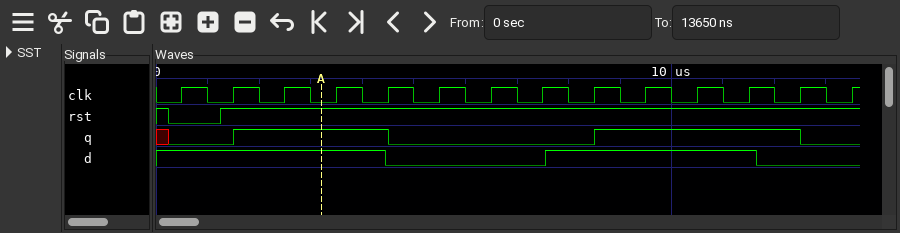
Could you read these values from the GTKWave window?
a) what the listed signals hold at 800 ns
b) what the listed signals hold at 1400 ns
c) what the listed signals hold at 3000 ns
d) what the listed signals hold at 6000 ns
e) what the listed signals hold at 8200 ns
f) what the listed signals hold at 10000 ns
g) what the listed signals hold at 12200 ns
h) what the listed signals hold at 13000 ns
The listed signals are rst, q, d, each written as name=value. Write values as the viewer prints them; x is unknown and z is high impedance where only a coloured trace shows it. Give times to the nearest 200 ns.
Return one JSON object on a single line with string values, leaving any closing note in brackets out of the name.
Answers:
{"what the listed signals hold at 800 ns": "rst=0, q=0, d=1", "what the listed signals hold at 1400 ns": "rst=1, q=0, d=1", "what the listed signals hold at 3000 ns": "rst=1, q=1, d=1", "what the listed signals hold at 6000 ns": "rst=1, q=0, d=0", "what the listed signals hold at 8200 ns": "rst=1, q=0, d=1", "what the listed signals hold at 10000 ns": "rst=1, q=1, d=1", "what the listed signals hold at 12200 ns": "rst=1, q=1, d=0", "what the listed signals hold at 13000 ns": "rst=1, q=0, d=0"}
